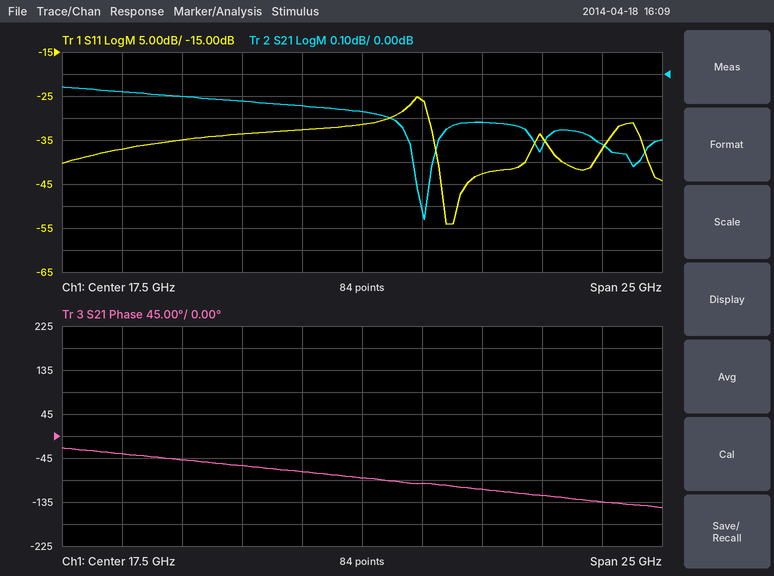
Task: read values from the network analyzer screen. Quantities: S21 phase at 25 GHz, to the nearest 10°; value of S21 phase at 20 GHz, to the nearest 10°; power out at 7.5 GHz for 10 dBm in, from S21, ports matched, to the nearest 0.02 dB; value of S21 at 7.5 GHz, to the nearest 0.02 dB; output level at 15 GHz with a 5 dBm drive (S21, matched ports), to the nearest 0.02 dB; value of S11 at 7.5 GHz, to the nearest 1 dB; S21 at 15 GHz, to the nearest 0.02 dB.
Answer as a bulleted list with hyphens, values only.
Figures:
- -120°
- -100°
- 9.92 dBm
- -0.08 dB
- 4.86 dBm
- -37 dB
- -0.14 dB
